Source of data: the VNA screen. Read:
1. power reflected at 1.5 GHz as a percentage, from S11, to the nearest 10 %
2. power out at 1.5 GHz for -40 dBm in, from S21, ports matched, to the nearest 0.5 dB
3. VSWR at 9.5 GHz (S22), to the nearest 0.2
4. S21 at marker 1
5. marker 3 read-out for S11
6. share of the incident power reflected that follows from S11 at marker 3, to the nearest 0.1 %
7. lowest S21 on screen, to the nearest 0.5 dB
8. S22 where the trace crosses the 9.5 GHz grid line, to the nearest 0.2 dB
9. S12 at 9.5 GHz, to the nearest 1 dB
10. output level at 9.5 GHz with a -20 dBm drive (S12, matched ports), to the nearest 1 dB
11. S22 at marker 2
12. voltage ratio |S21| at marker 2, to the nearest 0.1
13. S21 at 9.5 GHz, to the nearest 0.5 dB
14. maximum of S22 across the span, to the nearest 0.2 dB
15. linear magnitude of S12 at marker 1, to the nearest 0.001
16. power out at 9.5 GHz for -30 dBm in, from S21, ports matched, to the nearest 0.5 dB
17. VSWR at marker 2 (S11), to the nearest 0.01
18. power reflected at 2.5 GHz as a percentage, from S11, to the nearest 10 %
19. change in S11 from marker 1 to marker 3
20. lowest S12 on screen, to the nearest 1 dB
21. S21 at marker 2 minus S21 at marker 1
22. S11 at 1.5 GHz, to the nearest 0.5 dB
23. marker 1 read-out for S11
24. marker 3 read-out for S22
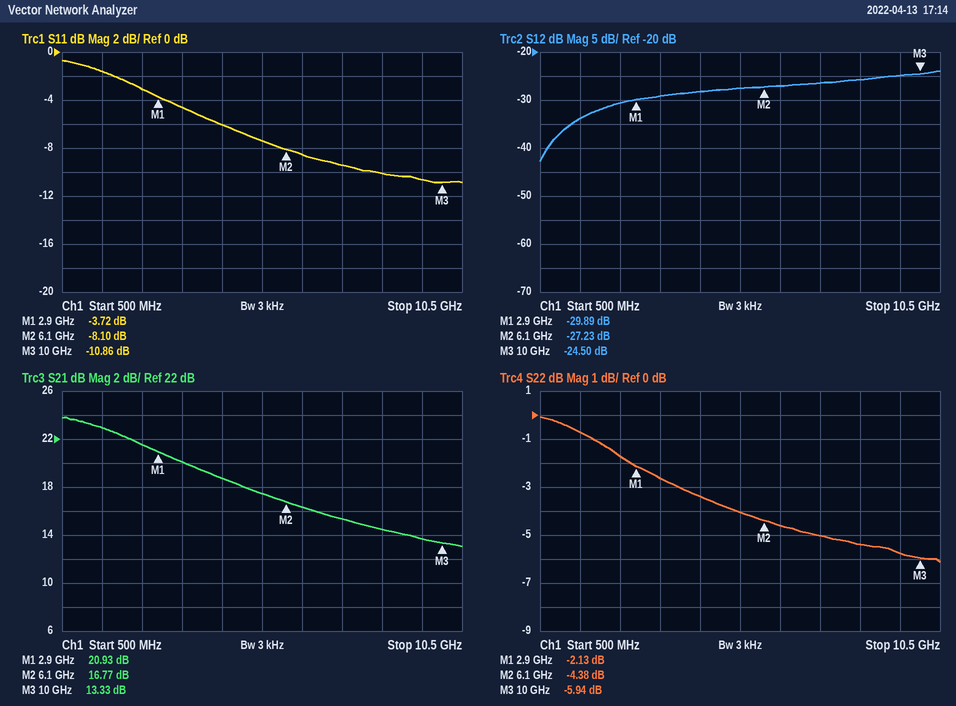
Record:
70 %
-17.0 dBm
3.2
20.93 dB
-10.86 dB
8.2 %
13.0 dB
-5.8 dB
-25 dB
-45 dBm
-4.38 dB
6.9
13.5 dB
0.0 dB
0.032
-16.5 dBm
2.30
50 %
-7.14 dB
-43 dB
-4.16 dB
-1.5 dB
-3.72 dB
-5.94 dB
